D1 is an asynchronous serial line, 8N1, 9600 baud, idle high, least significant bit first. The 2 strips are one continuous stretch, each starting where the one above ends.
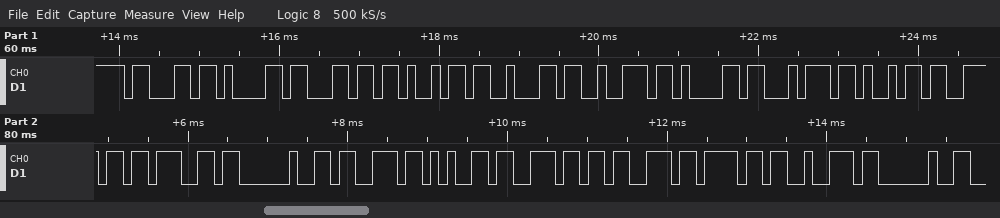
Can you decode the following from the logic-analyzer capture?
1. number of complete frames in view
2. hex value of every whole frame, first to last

19
63 61 6C 69 62 72 61 74 69 6E 67 20 73 65 6E 73 6F 72 20
